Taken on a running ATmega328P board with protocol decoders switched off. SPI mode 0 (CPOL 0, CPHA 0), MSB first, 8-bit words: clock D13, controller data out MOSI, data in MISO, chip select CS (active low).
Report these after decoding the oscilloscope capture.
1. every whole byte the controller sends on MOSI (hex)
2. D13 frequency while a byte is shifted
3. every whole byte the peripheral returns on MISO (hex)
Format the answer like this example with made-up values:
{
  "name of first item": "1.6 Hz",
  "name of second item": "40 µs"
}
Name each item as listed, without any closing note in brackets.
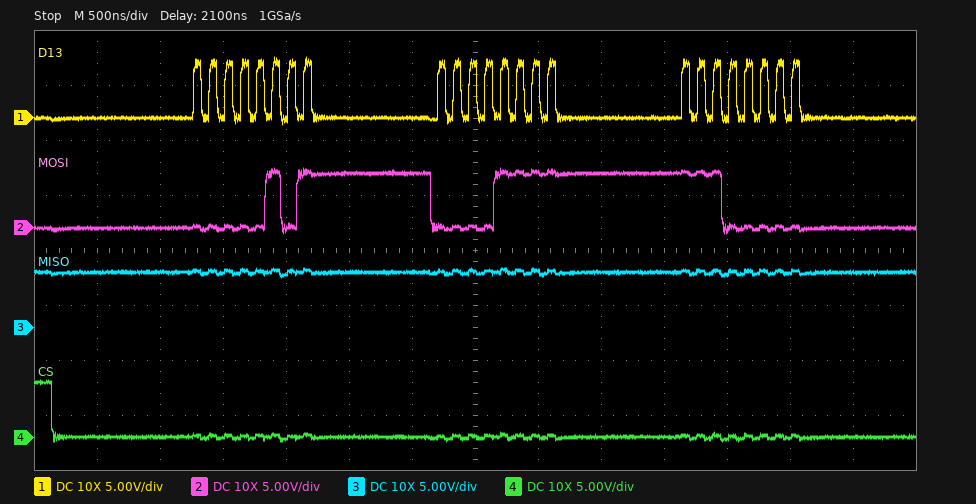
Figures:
{
  "every whole byte the controller sends on MOSI": "0x05 0x0F 0xE0",
  "D13 frequency while a byte is shifted": "8 MHz",
  "every whole byte the peripheral returns on MISO": "0xFF 0xFF 0xFF"
}
